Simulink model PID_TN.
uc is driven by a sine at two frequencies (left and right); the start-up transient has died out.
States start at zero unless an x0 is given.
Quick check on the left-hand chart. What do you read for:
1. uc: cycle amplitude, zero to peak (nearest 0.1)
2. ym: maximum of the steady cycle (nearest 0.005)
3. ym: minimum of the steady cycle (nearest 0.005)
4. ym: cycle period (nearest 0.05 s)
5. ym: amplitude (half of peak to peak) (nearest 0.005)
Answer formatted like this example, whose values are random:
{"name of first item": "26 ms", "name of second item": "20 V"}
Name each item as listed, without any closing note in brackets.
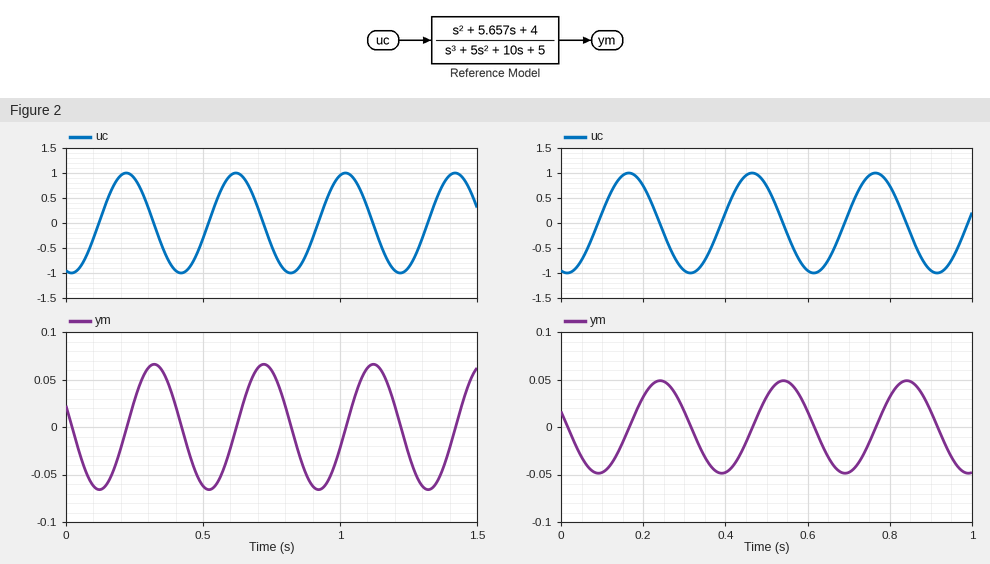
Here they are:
{"uc: cycle amplitude, zero to peak": "1.0", "ym: maximum of the steady cycle": "0.065", "ym: minimum of the steady cycle": "-0.065", "ym: cycle period": "0.40 s", "ym: amplitude (half of peak to peak)": "0.065"}
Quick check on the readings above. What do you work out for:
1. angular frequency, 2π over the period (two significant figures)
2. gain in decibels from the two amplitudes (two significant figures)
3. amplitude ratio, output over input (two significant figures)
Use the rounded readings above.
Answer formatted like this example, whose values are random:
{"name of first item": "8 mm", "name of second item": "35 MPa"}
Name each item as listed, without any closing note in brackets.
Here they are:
{"angular frequency, 2π over the period": "16 rad/s", "gain in decibels from the two amplitudes": "-24 dB", "amplitude ratio, output over input": "0.065"}
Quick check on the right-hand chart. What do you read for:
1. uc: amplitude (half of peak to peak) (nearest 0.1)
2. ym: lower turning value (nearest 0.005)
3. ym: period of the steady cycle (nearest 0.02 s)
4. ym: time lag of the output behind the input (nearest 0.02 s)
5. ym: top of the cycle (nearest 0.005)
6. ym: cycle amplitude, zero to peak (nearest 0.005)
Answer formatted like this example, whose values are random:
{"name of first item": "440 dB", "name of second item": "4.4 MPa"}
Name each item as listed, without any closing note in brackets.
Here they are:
{"uc: amplitude (half of peak to peak)": "1.0", "ym: lower turning value": "-0.050", "ym: period of the steady cycle": "0.30 s", "ym: time lag of the output behind the input": "0.08 s", "ym: top of the cycle": "0.050", "ym: cycle amplitude, zero to peak": "0.050"}
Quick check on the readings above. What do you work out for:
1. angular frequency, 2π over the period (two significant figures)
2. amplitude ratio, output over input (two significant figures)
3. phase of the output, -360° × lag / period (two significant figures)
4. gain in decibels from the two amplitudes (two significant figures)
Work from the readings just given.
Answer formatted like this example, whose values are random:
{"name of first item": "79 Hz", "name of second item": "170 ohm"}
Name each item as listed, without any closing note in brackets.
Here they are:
{"angular frequency, 2π over the period": "21 rad/s", "amplitude ratio, output over input": "0.050", "phase of the output, -360° × lag / period": "-96°", "gain in decibels from the two amplitudes": "-26 dB"}
